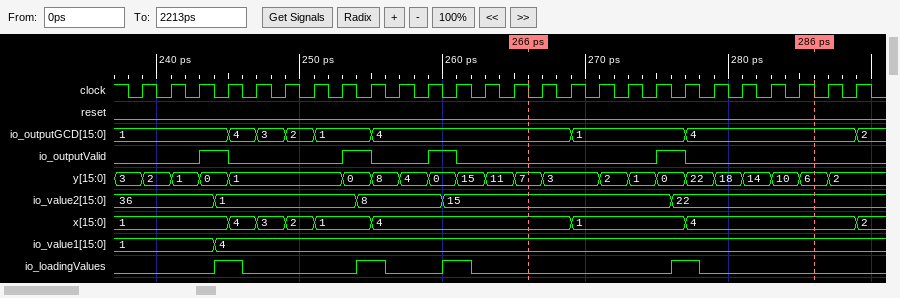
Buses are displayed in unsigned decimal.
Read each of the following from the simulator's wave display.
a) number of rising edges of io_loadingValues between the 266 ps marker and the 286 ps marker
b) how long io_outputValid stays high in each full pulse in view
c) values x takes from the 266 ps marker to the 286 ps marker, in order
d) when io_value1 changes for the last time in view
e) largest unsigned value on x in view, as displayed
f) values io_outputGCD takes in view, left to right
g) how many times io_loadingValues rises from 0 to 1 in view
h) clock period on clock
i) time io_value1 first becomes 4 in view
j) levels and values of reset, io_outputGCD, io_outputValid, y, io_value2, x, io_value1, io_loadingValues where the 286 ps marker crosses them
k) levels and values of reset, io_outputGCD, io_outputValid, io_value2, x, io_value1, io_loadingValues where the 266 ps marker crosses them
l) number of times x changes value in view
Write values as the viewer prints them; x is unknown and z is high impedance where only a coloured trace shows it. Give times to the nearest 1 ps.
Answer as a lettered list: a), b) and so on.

a) 1
b) 2 ps, 2 ps, 2 ps, 2 ps
c) 4, 1, 4
d) 244 ps
e) 4
f) 1, 4, 3, 2, 1, 4, 1, 4, 2
g) 4
h) 2 ps
i) 244 ps
j) reset=0, io_outputGCD=4, io_outputValid=0, y=6, io_value2=22, x=4, io_value1=4, io_loadingValues=0
k) reset=0, io_outputGCD=4, io_outputValid=0, io_value2=15, x=4, io_value1=4, io_loadingValues=0
l) 8
